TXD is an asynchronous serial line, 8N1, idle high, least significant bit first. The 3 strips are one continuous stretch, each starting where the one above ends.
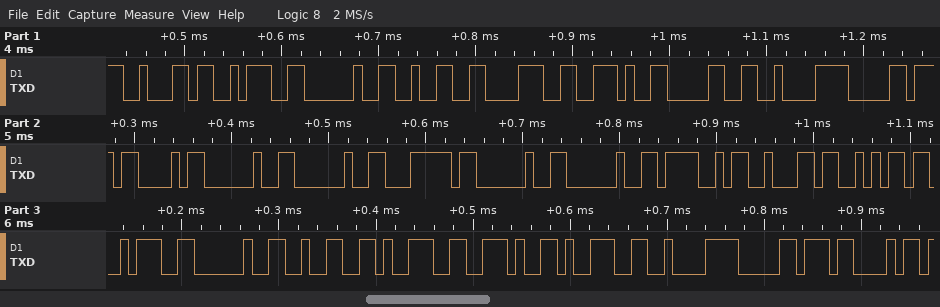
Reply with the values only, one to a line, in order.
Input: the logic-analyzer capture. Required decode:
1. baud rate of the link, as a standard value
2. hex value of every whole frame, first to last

115200 baud
62 3A 20 32 38 2E 30 C2 B0 43 20 20 7C 20 20 4F 62 6A 3A 20 32 39 2E 39 C2 B0 43
